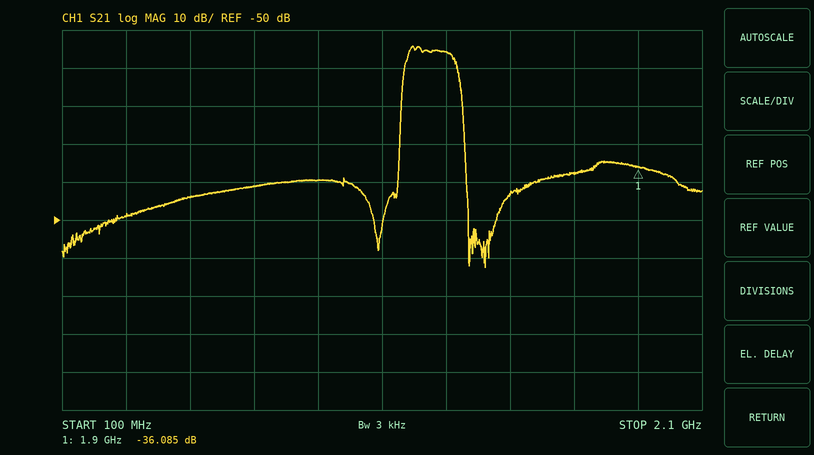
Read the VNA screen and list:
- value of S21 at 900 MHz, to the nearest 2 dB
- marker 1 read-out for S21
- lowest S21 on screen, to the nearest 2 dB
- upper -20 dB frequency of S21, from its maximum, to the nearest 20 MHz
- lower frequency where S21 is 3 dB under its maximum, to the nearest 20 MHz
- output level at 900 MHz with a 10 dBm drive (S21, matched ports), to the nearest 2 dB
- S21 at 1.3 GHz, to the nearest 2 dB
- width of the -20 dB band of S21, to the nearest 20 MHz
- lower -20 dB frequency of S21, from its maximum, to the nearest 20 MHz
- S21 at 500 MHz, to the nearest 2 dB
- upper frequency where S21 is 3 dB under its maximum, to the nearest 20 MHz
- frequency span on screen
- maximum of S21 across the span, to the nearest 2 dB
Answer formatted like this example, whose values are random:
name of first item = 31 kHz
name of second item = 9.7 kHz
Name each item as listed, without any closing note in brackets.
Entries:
value of S21 at 900 MHz, to the nearest 2 dB = -40 dB
marker 1 read-out for S21 = -36.085 dB
lowest S21 on screen, to the nearest 2 dB = -62 dB
upper -20 dB frequency of S21, from its maximum, to the nearest 20 MHz = 1.36 GHz
lower frequency where S21 is 3 dB under its maximum, to the nearest 20 MHz = 1.18 GHz
output level at 900 MHz with a 10 dBm drive (S21, matched ports), to the nearest 2 dB = -30 dBm
S21 at 1.3 GHz, to the nearest 2 dB = -6 dB
width of the -20 dB band of S21, to the nearest 20 MHz = 200 MHz
lower -20 dB frequency of S21, from its maximum, to the nearest 20 MHz = 1.16 GHz
S21 at 500 MHz, to the nearest 2 dB = -44 dB
upper frequency where S21 is 3 dB under its maximum, to the nearest 20 MHz = 1.32 GHz
frequency span on screen = 2 GHz
maximum of S21 across the span, to the nearest 2 dB = -4 dB
